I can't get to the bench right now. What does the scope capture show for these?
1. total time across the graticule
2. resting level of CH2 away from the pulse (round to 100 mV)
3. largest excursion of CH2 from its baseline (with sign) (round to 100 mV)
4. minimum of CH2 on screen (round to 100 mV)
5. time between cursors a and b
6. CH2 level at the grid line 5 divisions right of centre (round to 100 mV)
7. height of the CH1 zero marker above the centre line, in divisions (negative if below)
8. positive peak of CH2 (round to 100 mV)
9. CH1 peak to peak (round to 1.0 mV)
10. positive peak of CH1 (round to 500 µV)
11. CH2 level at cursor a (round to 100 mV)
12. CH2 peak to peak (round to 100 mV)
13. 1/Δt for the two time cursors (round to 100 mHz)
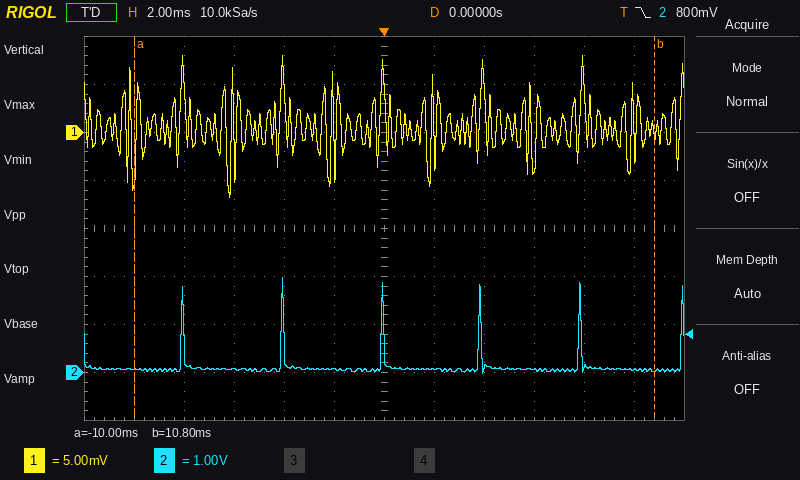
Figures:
24 ms
100 mV
+1.9 V
0.0 V
20.8 ms
100 mV
+2.0 div
2.0 V
15.0 mV
8.0 mV
100 mV
2.0 V
48.1 Hz
